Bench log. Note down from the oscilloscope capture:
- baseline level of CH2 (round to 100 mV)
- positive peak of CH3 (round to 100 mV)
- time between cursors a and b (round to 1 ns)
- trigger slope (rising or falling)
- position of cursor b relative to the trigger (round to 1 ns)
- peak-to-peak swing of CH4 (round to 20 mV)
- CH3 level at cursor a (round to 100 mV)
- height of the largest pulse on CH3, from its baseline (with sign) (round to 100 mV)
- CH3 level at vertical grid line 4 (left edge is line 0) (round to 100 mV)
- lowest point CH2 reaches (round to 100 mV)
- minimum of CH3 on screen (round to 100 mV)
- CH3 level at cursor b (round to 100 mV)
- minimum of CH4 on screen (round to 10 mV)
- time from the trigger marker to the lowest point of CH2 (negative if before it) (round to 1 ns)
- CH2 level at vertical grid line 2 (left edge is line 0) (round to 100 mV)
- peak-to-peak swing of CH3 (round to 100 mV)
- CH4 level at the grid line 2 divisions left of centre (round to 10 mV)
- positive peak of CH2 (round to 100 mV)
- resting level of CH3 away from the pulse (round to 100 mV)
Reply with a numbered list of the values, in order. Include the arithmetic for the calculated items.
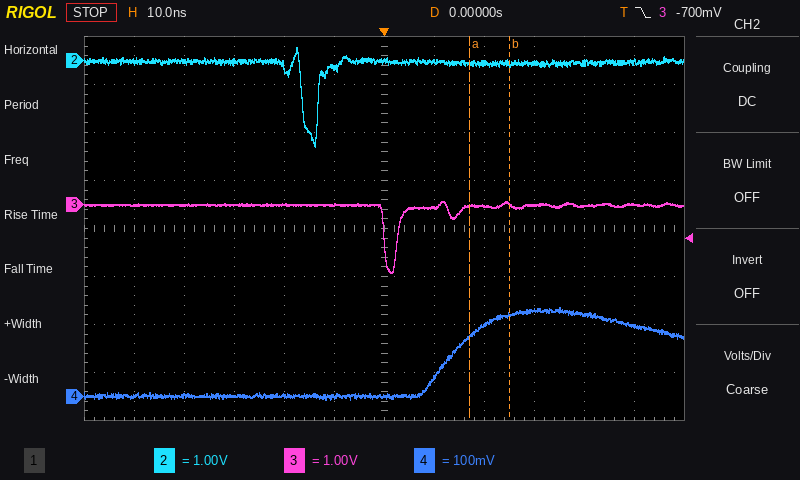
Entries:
1. 0.0 V
2. 100 mV
3. 8 ns
4. falling
5. +25 ns
6. 200 mV
7. 0.0 V
8. -1.4 V − (0.0 V) = -1.4 V
9. 0.0 V
10. -1.8 V
11. -1.4 V
12. 0.0 V
13. -10 mV
14. -14 ns
15. 0.0 V
16. 100 mV − (-1.4 V) = 1.5 V
17. 0 mV
18. 300 mV
19. 0.0 V
